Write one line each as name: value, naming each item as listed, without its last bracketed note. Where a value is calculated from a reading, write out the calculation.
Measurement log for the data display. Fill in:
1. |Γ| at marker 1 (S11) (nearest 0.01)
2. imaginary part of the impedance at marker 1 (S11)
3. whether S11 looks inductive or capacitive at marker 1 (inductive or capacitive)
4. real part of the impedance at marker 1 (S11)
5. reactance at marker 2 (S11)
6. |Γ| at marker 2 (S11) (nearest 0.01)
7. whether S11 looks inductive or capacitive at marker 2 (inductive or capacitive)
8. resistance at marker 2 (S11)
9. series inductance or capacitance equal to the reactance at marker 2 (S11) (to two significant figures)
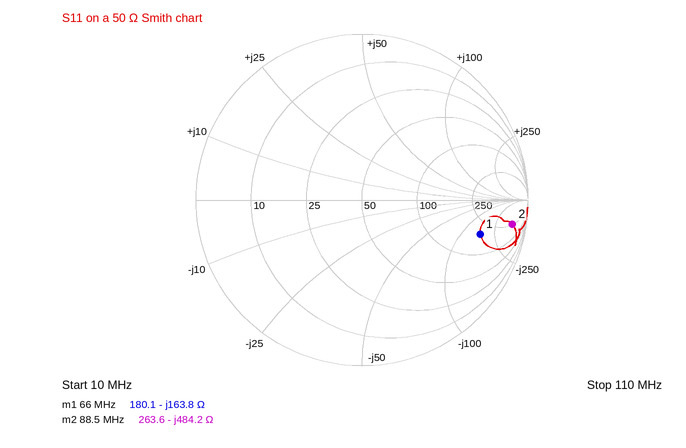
|Γ| at marker 1 (S11): 0.74
imaginary part of the impedance at marker 1: -163.8 Ω
whether S11 looks inductive or capacitive at marker 1: capacitive
real part of the impedance at marker 1: 180.1 Ω
reactance at marker 2: -484.2 Ω
|Γ| at marker 2 (S11): 0.92
whether S11 looks inductive or capacitive at marker 2: capacitive
resistance at marker 2: 263.6 Ω
series inductance or capacitance equal to the reactance at marker 2 (S11): C = 1/(2π × 88.5 MHz × 484.2 Ω) ≈ 3.7 pF
